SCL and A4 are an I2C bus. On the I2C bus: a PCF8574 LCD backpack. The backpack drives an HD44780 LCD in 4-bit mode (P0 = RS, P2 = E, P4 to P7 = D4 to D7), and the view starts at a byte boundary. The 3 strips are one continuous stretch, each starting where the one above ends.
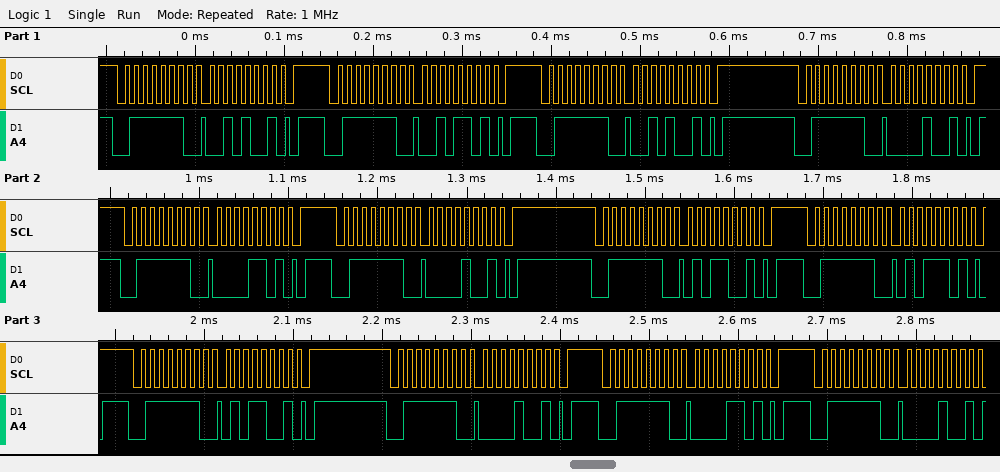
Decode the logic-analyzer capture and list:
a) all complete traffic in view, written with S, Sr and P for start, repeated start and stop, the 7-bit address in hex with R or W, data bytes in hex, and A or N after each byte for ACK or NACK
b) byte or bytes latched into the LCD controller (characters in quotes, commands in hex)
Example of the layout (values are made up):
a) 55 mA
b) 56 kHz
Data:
a) S 3FW A 29 A P S 3FW A 2D A P S 3FW A 29 A P S 3FW A 09 A P S 3FW A 0D A P S 3FW A 09 A P S 3FW A 59 A P S 3FW A 5D A P S 3FW A 59 A P S 3FW A 09 A P S 3FW A 0D A P S 3FW A 09 A
b) ' ' 'P'
